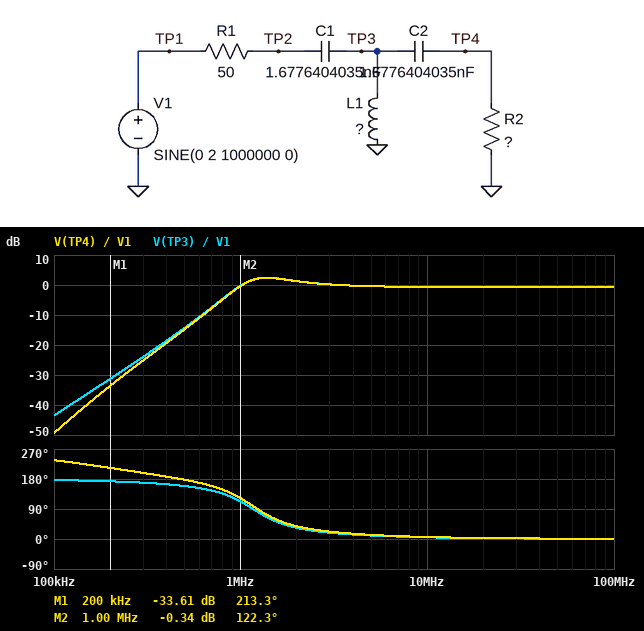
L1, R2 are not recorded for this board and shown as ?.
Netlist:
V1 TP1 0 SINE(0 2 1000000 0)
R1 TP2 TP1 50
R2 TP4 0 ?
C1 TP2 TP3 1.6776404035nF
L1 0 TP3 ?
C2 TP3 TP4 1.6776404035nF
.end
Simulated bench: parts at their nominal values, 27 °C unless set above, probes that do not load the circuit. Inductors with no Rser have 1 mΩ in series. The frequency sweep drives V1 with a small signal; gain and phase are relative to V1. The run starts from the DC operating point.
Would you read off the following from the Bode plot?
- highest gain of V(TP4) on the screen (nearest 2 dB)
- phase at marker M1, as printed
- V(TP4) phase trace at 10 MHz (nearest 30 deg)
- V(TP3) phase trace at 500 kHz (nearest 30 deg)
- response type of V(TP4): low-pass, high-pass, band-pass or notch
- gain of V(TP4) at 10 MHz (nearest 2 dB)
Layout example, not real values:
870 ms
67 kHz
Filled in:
2 dB
213.3 deg
0 deg
150 deg
high-pass
0 dB
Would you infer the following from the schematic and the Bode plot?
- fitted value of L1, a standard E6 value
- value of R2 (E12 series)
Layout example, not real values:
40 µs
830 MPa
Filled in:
10 µH
560 Ω
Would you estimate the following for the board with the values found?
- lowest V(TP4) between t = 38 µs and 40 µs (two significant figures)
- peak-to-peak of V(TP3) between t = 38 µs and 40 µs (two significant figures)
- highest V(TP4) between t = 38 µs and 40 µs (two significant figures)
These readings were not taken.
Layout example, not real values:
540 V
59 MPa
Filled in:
-1.9 V
3.9 V
1.9 V
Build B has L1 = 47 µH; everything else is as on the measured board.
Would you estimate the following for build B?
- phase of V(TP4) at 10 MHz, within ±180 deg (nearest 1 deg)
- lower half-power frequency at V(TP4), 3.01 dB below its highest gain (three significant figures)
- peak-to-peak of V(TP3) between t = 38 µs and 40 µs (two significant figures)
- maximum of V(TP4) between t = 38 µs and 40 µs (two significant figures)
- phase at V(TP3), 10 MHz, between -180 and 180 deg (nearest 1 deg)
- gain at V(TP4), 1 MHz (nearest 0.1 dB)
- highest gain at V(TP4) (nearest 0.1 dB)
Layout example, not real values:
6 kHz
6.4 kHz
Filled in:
3 deg
447 kHz
4.7 V
2.3 V
2 deg
1.2 dB
4.5 dB
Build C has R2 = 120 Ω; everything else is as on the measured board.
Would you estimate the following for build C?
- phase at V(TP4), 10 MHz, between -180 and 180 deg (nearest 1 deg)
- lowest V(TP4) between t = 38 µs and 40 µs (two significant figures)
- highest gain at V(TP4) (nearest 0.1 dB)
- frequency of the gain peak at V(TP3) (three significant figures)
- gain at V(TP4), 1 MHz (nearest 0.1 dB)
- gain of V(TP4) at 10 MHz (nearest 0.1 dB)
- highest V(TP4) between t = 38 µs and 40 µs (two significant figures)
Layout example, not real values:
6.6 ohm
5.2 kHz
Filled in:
10 deg
-1.4 V
-2.2 dB
1.10 MHz
-2.8 dB
-3.0 dB
1.4 V
